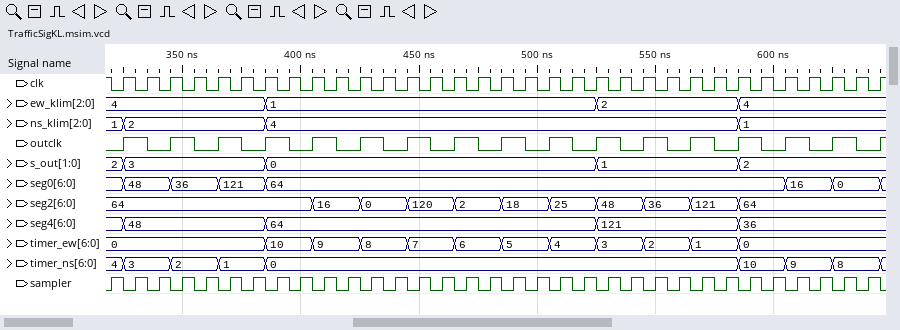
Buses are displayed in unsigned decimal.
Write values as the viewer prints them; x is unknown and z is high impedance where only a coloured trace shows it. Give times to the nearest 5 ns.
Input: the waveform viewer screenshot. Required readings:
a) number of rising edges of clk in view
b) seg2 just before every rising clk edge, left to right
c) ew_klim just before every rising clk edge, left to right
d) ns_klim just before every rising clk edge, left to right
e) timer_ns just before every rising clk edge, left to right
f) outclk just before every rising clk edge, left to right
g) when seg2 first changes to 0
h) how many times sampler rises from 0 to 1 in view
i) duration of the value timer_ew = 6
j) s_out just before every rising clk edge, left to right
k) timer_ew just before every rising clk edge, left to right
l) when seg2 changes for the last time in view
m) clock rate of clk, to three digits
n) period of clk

33
64, 64, 64, 64, 64, 64, 64, 64, 64, 16, 16, 0, 0, 120, 120, 2, 2, 18, 18, 25, 25, 48, 48, 36, 36, 121, 121, 64, 64, 64, 64, 64, 64
4, 4, 4, 4, 4, 4, 4, 1, 1, 1, 1, 1, 1, 1, 1, 1, 1, 1, 1, 1, 1, 2, 2, 2, 2, 2, 2, 4, 4, 4, 4, 4, 4
1, 2, 2, 2, 2, 2, 2, 4, 4, 4, 4, 4, 4, 4, 4, 4, 4, 4, 4, 4, 4, 4, 4, 4, 4, 4, 4, 1, 1, 1, 1, 1, 1
4, 3, 3, 2, 2, 1, 1, 0, 0, 0, 0, 0, 0, 0, 0, 0, 0, 0, 0, 0, 0, 0, 0, 0, 0, 0, 0, 10, 10, 9, 9, 8, 8
0 1 0 1 0 1 0 1 0 1 0 1 0 1 0 1 0 1 0 1 0 1 0 1 0 1 0 1 0 1 0 1 0
425 ns
33
20 ns
2, 3, 3, 3, 3, 3, 3, 0, 0, 0, 0, 0, 0, 0, 0, 0, 0, 0, 0, 0, 0, 1, 1, 1, 1, 1, 1, 2, 2, 2, 2, 2, 2
0, 0, 0, 0, 0, 0, 0, 10, 10, 9, 9, 8, 8, 7, 7, 6, 6, 5, 5, 4, 4, 3, 3, 2, 2, 1, 1, 0, 0, 0, 0, 0, 0
585 ns
100 MHz
10 ns
